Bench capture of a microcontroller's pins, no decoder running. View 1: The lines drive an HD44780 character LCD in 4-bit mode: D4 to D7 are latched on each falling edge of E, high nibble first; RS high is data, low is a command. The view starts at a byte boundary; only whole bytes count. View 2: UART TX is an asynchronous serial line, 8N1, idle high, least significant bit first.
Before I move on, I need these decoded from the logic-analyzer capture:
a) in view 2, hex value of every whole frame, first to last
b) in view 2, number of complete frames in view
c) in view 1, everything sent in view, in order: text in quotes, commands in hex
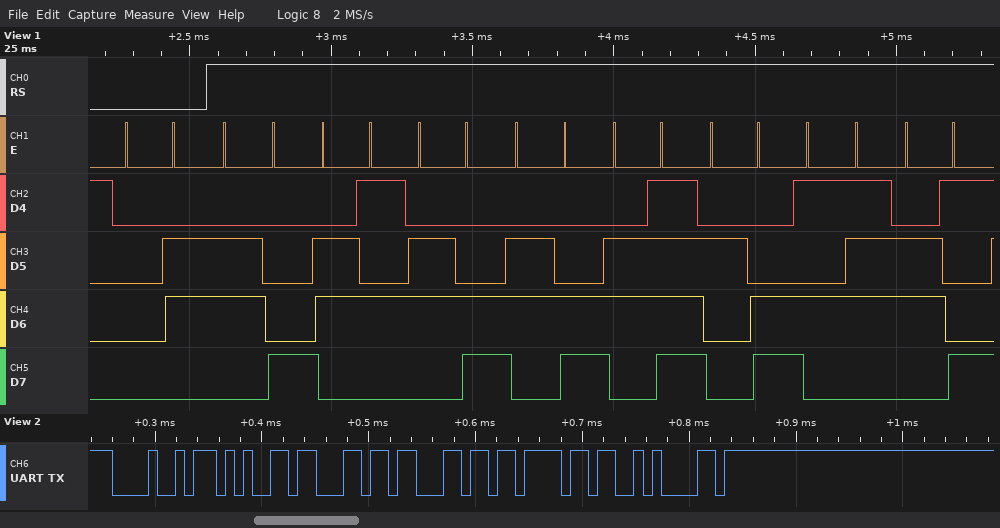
48 65 6C 6C 6F 0A FF
7
0x06 "hello,Wi"
